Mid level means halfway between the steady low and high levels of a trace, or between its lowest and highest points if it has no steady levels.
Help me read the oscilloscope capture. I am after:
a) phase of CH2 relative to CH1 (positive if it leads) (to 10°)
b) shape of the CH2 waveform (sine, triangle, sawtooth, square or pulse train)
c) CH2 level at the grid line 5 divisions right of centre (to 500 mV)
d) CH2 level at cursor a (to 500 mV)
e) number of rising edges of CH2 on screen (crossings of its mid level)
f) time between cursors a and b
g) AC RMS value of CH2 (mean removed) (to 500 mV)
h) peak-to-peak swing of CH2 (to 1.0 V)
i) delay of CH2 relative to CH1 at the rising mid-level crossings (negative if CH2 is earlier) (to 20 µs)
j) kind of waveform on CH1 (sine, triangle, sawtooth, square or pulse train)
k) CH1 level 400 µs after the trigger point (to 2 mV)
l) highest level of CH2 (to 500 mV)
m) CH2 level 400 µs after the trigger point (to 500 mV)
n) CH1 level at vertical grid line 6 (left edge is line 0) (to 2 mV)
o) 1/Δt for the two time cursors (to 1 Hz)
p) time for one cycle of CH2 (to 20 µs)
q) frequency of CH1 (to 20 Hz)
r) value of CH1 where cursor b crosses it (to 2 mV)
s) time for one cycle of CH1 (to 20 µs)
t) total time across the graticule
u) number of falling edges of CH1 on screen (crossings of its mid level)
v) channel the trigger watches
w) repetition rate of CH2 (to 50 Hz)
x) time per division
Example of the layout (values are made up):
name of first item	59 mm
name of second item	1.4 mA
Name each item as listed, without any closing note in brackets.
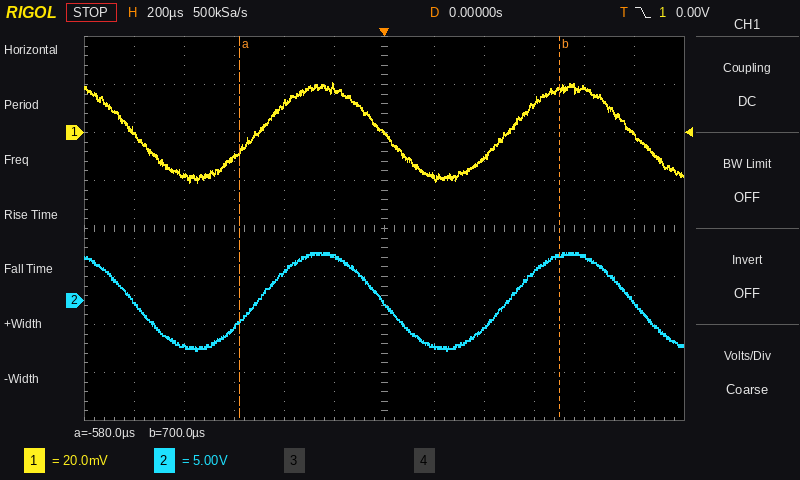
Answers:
phase of CH2 relative to CH1 (positive if it leads)	0°
shape of the CH2 waveform	sine
CH2 level at the grid line 5 divisions right of centre	0.0 V
CH2 level at cursor a	-2.0 V
number of rising edges of CH2 on screen	2
time between cursors a and b	1.28 ms
AC RMS value of CH2 (mean removed)	3.5 V
peak-to-peak swing of CH2	10.0 V
delay of CH2 relative to CH1 at the rising mid-level crossings (negative if CH2 is earlier)	0 µs
kind of waveform on CH1	sine
CH1 level 400 µs after the trigger point	-10 mV
highest level of CH2	5.0 V
CH2 level 400 µs after the trigger point	-3.0 V
CH1 level at vertical grid line 6 (left edge is line 0)	0 mV
1/Δt for the two time cursors	781 Hz
time for one cycle of CH2	1.00 ms
frequency of CH1	1.00 kHz
value of CH1 where cursor b crosses it	18 mV
time for one cycle of CH1	1.00 ms
total time across the graticule	2.4 ms
number of falling edges of CH1 on screen	3
channel the trigger watches	CH1
repetition rate of CH2	1.00 kHz
time per division	200 µs
